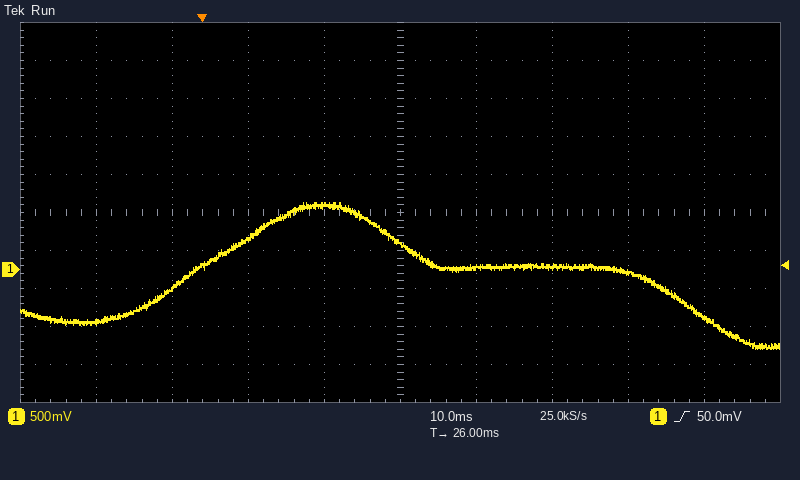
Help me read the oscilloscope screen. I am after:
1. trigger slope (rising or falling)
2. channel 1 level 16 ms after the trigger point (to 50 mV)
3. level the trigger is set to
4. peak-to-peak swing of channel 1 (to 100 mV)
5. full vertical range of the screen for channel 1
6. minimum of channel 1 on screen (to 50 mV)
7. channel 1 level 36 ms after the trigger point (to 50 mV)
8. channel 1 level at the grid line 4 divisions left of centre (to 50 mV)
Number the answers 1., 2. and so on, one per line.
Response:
1. rising
2. 850 mV
3. 50.0 mV
4. 1.90 V
5. 5 V
6. -1.05 V
7. 50 mV
8. -700 mV
